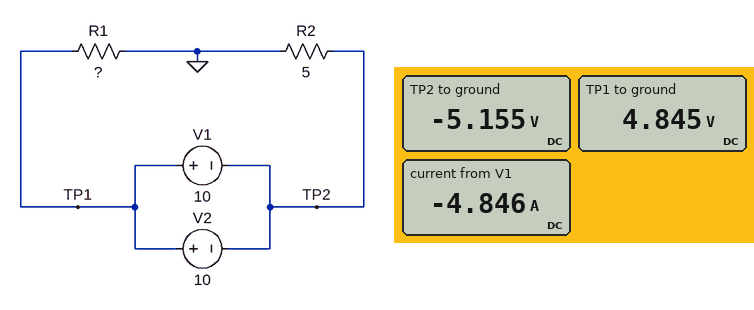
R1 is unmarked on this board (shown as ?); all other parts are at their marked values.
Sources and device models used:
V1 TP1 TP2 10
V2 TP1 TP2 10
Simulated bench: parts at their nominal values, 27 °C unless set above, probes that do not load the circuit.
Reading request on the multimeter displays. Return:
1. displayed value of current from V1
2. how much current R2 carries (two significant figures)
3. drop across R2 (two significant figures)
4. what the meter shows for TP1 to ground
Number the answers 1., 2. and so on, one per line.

1. -4.846 A
2. 1.0 A
3. 5.2 V
4. 4.845 V
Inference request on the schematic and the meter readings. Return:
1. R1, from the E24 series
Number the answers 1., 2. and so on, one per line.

1. 4.7 Ω
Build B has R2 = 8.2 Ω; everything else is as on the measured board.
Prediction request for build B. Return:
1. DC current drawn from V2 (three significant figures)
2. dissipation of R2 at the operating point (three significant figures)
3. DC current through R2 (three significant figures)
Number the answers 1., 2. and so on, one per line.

1. 4.42 A
2. 4.93 W
3. 775 mA
